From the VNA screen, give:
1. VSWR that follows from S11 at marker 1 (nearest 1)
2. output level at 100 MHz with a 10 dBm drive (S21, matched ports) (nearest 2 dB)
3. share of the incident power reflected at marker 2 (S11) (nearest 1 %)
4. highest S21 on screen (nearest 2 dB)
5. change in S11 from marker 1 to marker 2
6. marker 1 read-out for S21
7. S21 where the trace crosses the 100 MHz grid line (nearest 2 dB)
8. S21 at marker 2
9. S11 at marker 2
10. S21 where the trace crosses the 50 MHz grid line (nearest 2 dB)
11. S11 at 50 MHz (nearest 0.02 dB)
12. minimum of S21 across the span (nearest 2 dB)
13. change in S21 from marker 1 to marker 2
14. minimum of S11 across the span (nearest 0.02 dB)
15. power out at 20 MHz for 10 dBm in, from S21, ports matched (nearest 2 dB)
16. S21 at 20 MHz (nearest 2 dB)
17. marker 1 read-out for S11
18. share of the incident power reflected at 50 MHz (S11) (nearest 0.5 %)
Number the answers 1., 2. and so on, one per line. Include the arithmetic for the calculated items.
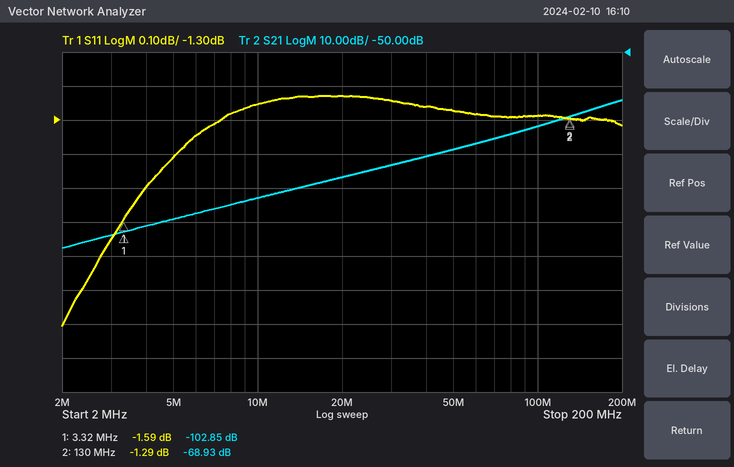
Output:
1. (1 + 0.8327)/(1 − 0.8327) ≈ 11
2. 10 dBm + (-72 dB) = -62 dBm
3. 10^(-1.29/10) ≈ 74 %
4. -64 dB
5. -1.29 − (-1.59) = 0.30 dB
6. -102.85 dB
7. -72 dB
8. -68.93 dB
9. -1.29 dB
10. -78 dB
11. -1.28 dB
12. -108 dB
13. -68.93 − (-102.85) = 33.92 dB
14. -1.90 dB
15. 10 dBm + (-86 dB) = -76 dBm
16. -86 dB
17. -1.59 dB
18. 10^(-1.28/10) ≈ 74.5 %
